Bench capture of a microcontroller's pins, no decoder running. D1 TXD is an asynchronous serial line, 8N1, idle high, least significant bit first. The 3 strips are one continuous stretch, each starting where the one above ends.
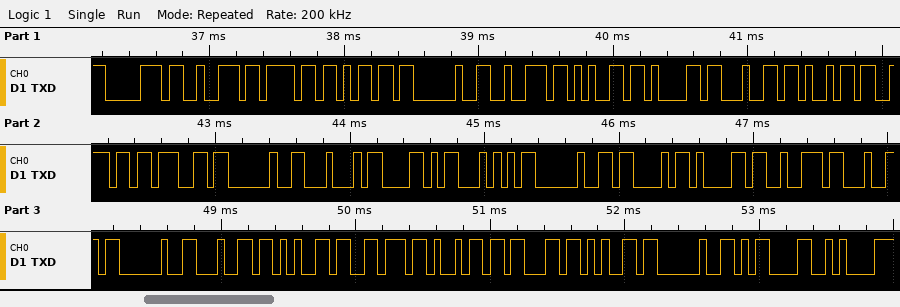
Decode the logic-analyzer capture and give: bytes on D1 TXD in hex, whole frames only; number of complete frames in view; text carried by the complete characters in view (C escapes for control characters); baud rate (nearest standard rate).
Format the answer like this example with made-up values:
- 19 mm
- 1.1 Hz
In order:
- 0x70 0x72 0x6F 0x6D 0x20 0x72 0x65 0x61 0x64 0x69 0x6E 0x67 0x20 0x44 0x58 0x54 0x20 0x43 0x61 0x72 0x64 0x20 0x64 0x65 0x76 0x69 0x63 0x65 0x20 0x0D 0x0A
- 31
- "prom reading DXT Card device \r\n"
- 19200 baud
